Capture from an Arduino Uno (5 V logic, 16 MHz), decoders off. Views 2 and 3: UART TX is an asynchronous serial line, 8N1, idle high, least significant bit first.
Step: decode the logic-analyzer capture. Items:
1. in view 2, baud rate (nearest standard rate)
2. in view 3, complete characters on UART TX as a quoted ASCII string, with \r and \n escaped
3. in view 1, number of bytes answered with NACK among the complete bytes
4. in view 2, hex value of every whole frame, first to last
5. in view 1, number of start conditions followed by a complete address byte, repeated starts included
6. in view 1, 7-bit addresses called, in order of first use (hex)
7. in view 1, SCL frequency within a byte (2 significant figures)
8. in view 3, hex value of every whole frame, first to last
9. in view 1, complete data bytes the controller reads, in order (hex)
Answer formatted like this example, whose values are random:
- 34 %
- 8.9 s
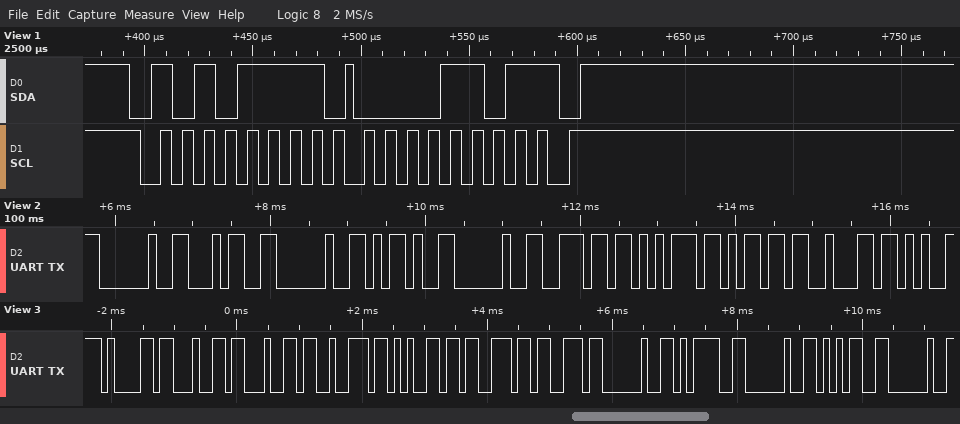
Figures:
- 9600 baud
- "address = 5 "
- 1
- 20 34 20 2D 20 6E 75 6D 62
- 1
- 0x57
- 100 kHz
- 61 64 64 72 65 73 73 20 3D 20 35 20
- 0D
